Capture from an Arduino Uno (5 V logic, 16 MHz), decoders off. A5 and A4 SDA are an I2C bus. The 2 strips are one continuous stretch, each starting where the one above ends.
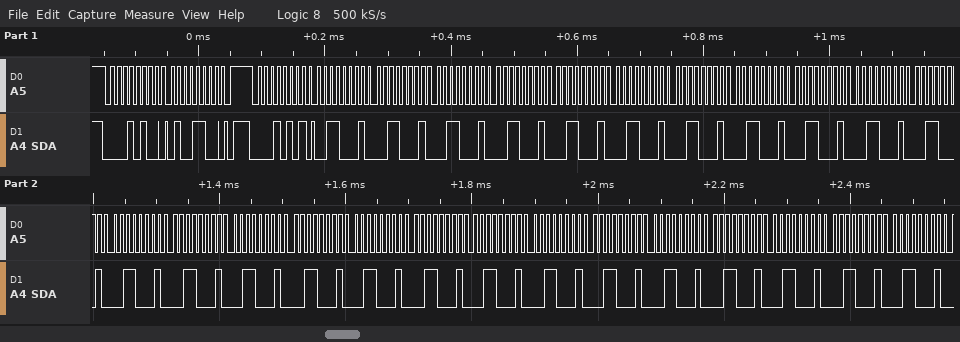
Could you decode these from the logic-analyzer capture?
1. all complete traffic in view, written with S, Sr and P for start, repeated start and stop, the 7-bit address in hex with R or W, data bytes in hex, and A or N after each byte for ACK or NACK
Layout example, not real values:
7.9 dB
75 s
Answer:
S 0AW A 4C A P S 0AR A 31 A 31 A 31 A 31 A 31 A 31 A 31 A 31 A 31 A 31 A 31 A 31 A 31 A 31 A 31 A 31 A 31 A 31 A 31 A 31 A 31 A 31 A 31 A 31 A 31 A
